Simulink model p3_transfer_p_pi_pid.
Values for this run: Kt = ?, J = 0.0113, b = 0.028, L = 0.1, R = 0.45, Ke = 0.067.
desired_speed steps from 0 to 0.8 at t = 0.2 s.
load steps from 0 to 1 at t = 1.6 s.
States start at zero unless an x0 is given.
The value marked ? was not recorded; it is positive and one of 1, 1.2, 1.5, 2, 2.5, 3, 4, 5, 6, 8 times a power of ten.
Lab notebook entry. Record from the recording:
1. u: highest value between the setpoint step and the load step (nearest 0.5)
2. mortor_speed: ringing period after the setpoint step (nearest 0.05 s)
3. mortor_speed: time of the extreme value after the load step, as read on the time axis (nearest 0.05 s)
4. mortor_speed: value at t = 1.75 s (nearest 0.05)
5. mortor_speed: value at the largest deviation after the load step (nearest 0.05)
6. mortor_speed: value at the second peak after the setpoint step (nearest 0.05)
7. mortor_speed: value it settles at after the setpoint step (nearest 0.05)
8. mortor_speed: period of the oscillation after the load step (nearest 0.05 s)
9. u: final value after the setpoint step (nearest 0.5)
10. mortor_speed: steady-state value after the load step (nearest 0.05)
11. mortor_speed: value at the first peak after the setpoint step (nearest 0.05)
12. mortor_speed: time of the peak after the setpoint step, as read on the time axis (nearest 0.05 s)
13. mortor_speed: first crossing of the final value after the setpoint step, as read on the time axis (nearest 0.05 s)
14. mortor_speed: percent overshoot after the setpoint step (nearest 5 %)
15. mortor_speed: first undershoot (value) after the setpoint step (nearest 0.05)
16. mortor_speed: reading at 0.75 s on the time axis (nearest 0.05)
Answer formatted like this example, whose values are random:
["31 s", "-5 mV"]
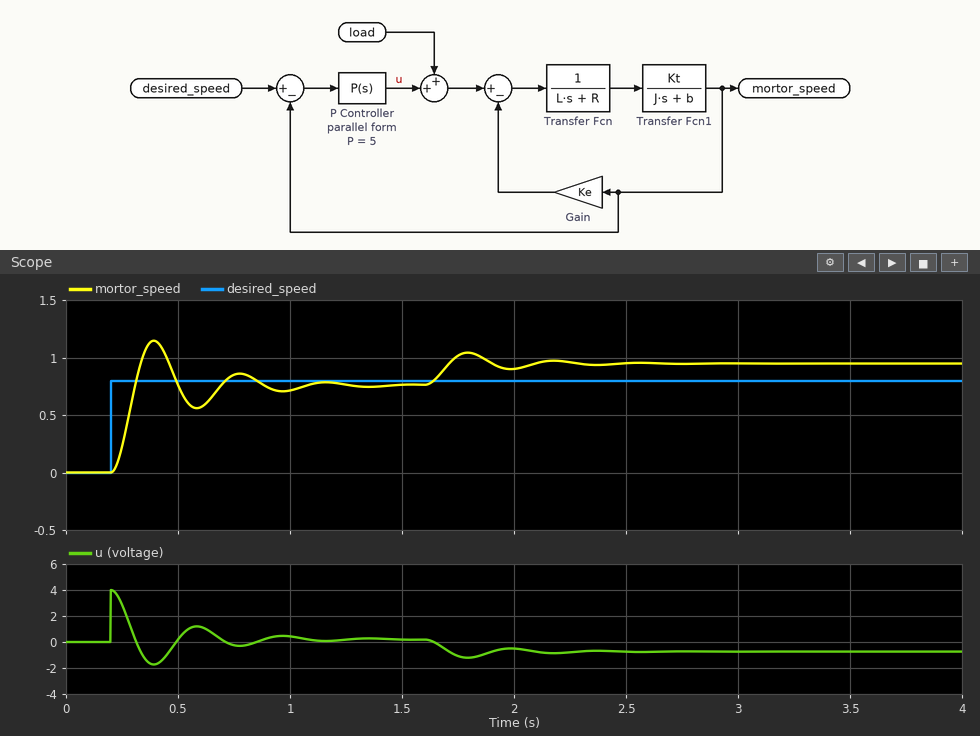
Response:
["4.0", "0.40 s", "1.80 s", "1.00", "1.05", "0.85", "0.75", "0.40 s", "0.0", "0.95", "1.15", "0.40 s", "0.30 s", "50 %", "0.55", "0.85"]
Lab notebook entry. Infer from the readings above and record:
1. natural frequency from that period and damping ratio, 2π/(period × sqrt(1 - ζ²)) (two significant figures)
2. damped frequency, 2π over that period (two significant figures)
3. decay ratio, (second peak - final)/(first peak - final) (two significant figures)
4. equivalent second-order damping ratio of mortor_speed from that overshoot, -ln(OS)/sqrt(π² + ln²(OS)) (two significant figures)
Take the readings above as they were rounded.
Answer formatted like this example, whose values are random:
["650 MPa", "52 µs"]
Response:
["16 rad/s", "16 rad/s", "0.25", "0.22"]
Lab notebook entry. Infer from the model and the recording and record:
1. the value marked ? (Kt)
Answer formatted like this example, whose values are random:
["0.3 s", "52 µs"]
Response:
["0.06"]
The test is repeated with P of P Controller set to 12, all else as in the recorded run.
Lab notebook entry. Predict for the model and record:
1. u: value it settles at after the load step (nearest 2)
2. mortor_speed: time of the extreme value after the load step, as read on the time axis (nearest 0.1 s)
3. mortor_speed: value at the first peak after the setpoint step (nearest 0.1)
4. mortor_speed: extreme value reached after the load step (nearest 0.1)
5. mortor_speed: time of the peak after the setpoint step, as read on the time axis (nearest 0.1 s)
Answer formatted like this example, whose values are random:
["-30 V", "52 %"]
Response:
["0", "1.7 s", "1.3", "0.9", "0.3 s"]
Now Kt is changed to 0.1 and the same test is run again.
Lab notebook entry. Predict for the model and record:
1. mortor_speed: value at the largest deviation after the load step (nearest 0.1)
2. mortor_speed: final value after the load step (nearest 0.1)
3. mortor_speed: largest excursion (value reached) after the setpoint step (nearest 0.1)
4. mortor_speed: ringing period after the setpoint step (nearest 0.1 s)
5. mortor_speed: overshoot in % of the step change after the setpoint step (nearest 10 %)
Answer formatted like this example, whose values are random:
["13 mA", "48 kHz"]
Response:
["1.1", "1.0", "1.2", "0.3 s", "60 %"]
